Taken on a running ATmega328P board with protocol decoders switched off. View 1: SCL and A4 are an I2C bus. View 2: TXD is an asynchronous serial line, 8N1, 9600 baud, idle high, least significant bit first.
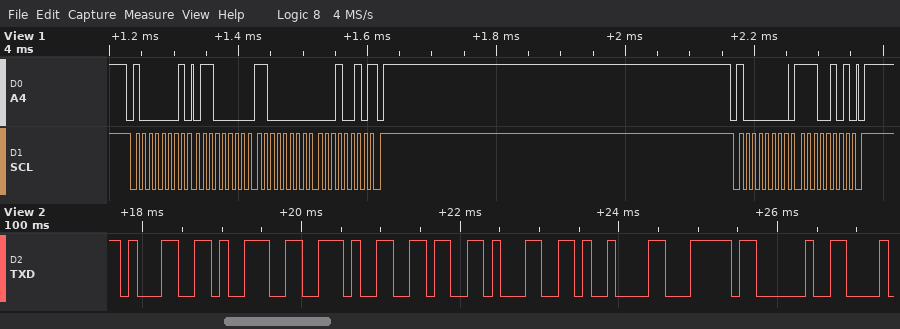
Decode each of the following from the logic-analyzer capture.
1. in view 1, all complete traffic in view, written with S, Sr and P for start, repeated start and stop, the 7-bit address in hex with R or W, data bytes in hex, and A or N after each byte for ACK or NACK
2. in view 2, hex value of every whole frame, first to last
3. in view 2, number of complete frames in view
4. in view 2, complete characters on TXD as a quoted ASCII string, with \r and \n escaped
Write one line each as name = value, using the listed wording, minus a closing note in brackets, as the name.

in view 1, all complete traffic in view, written with S, Sr and P for start, repeated start and stop, the 7-bit address in hex with R or W, data bytes in hex, and A or N after each byte for ACK or NACK = S 40R A 60 A C0 A 12 N P S 40W A E5 A P
in view 2, hex value of every whole frame, first to last = 0x31 0x39 0x2E 0x36 0x31 0x09 0x7C 0x20
in view 2, number of complete frames in view = 8
in view 2, complete characters on TXD as a quoted ASCII string, with \r and \n escaped = "19.61\t| "
